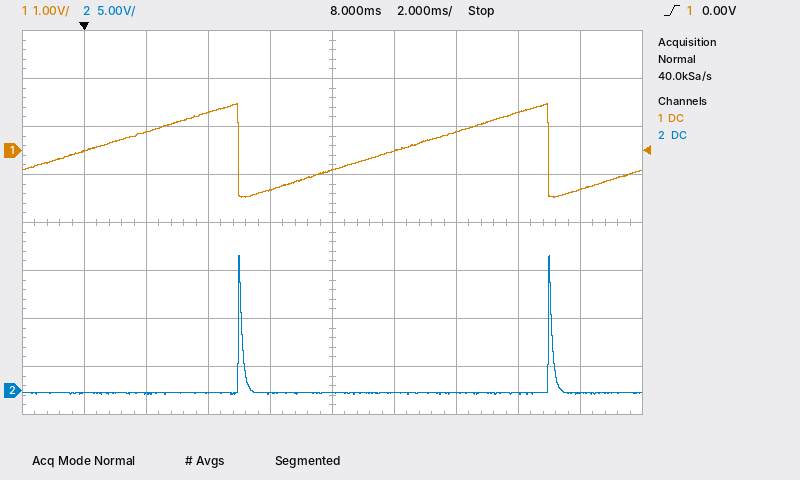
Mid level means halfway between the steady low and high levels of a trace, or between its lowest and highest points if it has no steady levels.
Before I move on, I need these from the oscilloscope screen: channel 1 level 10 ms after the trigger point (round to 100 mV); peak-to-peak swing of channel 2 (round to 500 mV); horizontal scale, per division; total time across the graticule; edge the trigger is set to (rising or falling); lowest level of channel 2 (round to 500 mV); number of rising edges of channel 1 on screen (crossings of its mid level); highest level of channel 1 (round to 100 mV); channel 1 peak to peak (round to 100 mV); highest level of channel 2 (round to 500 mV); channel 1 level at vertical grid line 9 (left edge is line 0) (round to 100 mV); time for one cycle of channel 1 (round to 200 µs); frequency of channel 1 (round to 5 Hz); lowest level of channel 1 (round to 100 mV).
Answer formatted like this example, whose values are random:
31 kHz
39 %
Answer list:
0.0 V
14.5 V
2 ms
20 ms
rising
-500 mV
2
1.0 V
2.0 V
14.0 V
-800 mV
10.0 ms
100 Hz
-1.0 V
